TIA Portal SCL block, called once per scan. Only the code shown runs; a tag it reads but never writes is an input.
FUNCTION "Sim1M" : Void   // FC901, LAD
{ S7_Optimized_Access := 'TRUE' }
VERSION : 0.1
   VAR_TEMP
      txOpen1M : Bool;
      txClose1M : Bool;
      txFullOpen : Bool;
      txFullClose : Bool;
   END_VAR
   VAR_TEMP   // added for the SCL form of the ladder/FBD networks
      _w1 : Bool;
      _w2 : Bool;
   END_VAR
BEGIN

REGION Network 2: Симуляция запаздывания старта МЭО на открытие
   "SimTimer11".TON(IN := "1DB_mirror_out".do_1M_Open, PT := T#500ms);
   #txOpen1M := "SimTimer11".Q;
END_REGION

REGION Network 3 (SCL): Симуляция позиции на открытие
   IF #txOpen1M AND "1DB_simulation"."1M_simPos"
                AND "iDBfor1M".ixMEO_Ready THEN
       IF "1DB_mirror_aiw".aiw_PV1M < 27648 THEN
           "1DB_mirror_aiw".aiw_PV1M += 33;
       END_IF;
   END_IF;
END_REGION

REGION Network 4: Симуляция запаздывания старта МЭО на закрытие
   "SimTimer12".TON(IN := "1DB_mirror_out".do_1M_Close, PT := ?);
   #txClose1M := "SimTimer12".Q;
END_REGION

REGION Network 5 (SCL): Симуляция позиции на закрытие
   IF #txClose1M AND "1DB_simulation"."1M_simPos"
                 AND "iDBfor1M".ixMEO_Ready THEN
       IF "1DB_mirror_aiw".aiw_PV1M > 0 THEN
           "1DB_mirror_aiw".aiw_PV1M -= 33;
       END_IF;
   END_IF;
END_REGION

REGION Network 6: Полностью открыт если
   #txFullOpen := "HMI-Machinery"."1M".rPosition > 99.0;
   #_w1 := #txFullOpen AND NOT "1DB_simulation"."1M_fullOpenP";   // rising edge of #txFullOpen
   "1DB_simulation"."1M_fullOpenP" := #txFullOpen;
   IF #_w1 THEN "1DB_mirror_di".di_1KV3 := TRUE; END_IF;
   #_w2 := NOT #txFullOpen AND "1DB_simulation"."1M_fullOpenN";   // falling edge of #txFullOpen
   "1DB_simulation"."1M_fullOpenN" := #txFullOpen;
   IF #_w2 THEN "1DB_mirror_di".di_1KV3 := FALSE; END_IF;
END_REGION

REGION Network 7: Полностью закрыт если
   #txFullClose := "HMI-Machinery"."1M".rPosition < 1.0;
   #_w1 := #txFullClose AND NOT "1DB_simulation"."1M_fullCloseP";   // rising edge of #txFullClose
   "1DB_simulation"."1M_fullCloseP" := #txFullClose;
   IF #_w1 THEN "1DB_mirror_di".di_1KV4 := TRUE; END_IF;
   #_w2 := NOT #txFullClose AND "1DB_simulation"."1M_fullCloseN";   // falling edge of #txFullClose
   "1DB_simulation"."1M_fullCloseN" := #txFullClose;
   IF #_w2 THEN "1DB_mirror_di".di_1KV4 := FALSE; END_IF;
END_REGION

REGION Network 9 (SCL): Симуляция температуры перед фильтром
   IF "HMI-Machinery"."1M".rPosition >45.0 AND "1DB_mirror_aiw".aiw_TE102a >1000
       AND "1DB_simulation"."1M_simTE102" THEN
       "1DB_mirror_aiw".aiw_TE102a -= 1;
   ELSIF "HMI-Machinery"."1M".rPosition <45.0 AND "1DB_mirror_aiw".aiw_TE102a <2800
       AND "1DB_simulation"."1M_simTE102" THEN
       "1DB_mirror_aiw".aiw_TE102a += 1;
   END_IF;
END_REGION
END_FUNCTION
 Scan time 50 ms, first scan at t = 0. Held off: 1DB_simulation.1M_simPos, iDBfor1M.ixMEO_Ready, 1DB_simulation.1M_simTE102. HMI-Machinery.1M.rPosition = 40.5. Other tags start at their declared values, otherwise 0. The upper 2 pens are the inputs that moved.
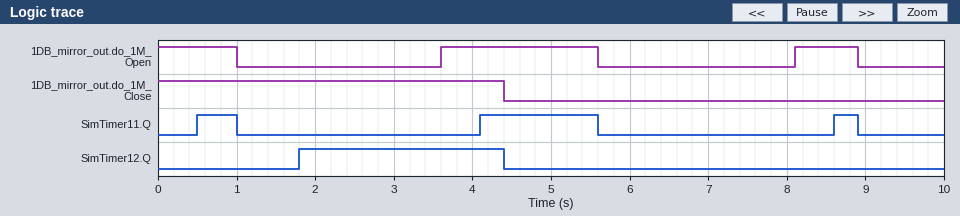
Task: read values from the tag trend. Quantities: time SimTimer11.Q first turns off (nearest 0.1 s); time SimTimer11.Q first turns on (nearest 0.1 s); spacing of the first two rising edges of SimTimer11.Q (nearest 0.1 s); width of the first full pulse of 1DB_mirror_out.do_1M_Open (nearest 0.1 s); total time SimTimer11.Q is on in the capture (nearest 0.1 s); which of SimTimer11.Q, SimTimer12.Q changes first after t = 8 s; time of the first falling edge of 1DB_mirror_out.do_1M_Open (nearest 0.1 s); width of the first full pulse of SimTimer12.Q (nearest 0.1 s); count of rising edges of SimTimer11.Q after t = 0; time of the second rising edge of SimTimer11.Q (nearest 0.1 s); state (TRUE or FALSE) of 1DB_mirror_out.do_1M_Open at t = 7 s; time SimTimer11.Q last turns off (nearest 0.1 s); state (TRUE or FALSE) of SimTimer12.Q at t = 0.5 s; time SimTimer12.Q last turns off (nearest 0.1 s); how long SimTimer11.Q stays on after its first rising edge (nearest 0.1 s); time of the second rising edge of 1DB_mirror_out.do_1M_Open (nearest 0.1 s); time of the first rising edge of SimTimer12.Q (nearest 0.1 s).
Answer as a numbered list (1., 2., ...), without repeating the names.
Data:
1. 1.0 s
2. 0.5 s
3. 3.6 s
4. 2.0 s
5. 2.3 s
6. SimTimer11.Q
7. 1.0 s
8. 2.6 s
9. 3
10. 4.1 s
11. FALSE
12. 8.9 s
13. FALSE
14. 4.4 s
15. 0.5 s
16. 8.1 s
17. 1.8 s
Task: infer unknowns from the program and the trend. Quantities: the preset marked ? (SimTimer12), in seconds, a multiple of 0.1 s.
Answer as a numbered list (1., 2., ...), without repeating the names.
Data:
1. 1.8 s
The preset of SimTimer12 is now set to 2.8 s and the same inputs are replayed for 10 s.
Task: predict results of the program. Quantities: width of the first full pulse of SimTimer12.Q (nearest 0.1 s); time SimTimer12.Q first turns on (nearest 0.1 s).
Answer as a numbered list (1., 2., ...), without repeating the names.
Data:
1. 1.6 s
2. 2.8 s
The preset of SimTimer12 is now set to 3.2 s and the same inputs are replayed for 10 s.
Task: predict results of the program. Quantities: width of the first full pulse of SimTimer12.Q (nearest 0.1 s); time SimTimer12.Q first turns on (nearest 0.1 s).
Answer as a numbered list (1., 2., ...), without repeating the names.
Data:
1. 1.2 s
2. 3.2 s
